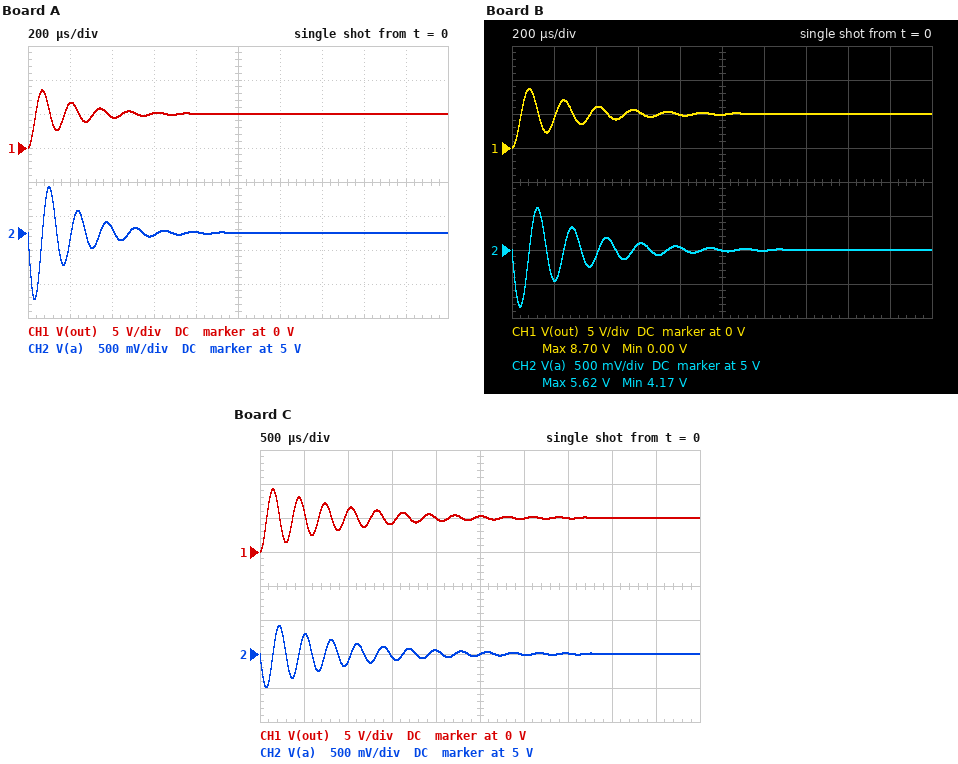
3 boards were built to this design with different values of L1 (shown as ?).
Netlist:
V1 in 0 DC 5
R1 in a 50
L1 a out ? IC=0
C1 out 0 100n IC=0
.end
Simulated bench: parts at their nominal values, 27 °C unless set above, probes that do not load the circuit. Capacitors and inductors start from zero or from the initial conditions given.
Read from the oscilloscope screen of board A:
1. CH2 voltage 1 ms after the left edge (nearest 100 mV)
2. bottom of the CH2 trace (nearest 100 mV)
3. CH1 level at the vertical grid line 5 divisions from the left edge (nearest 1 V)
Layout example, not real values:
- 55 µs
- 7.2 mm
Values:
- 5.0 V
- 4.0 V
- 5 V
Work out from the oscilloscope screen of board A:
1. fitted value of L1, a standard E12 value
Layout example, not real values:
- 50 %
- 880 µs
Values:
- 4.7 mH
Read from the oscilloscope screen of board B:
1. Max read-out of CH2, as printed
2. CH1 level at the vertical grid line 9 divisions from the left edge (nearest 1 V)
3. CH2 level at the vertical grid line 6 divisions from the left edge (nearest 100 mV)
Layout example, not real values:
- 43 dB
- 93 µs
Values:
- 5.62 V
- 5 V
- 5.0 V
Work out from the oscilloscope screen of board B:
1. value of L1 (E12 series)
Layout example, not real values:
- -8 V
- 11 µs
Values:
- 6.8 mH
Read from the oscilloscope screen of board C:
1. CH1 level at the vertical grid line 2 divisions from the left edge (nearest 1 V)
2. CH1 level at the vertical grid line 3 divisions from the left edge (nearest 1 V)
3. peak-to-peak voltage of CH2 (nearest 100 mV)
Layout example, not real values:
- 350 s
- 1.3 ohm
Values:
- 6 V
- 4 V
- 900 mV
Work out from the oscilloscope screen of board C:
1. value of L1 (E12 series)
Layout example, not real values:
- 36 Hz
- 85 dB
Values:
- 22 mH
